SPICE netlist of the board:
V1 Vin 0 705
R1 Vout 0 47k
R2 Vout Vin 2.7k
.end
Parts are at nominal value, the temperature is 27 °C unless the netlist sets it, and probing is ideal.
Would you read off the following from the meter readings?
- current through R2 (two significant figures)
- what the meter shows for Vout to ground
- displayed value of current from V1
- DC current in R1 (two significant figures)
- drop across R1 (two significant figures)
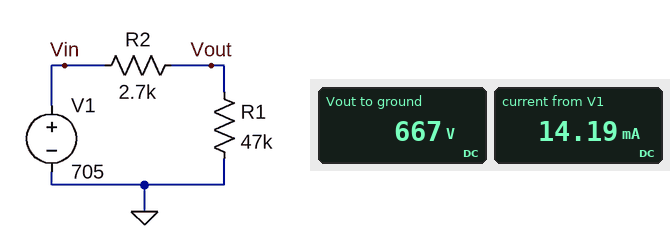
14 mA
667 V
14.19 mA
14 mA
670 V
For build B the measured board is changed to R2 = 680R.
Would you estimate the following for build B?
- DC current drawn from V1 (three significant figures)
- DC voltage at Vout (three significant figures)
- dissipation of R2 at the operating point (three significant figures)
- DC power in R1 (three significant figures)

14.8 mA
695 V
149 mW
10.3 W
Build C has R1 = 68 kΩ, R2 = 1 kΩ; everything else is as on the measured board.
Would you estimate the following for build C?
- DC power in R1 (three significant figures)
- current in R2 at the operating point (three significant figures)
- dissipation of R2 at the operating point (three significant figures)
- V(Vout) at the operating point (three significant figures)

7.10 W
10.2 mA
104 mW
695 V
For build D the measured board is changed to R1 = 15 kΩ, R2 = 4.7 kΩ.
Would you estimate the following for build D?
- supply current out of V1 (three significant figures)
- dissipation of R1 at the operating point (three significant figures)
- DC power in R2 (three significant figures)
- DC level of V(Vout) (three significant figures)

35.8 mA
19.2 W
6.02 W
537 V
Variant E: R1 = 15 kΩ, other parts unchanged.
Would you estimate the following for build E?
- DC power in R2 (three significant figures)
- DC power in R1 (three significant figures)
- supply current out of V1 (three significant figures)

4.28 W
23.8 W
39.8 mA
